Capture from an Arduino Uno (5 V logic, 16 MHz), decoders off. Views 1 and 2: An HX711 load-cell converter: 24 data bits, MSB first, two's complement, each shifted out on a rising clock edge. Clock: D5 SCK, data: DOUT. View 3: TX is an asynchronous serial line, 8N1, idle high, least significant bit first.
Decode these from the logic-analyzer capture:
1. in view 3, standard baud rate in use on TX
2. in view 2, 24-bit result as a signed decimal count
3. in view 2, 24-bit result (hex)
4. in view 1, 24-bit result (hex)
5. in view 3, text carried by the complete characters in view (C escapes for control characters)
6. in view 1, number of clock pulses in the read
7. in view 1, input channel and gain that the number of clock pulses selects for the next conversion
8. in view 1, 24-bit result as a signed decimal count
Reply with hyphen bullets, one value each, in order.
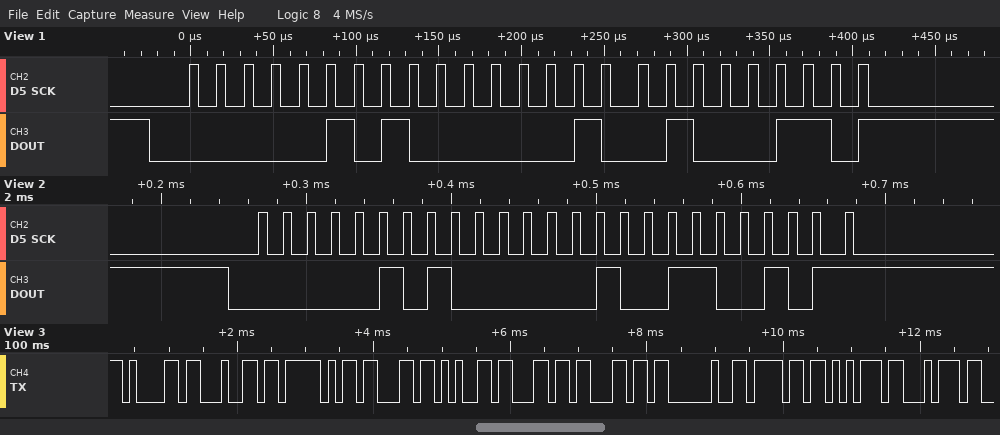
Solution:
- 9600 baud
- 328293
- 0x050265
- 0x050246
- "ad_cell out"
- 25
- channel A, gain 128
- 328262
